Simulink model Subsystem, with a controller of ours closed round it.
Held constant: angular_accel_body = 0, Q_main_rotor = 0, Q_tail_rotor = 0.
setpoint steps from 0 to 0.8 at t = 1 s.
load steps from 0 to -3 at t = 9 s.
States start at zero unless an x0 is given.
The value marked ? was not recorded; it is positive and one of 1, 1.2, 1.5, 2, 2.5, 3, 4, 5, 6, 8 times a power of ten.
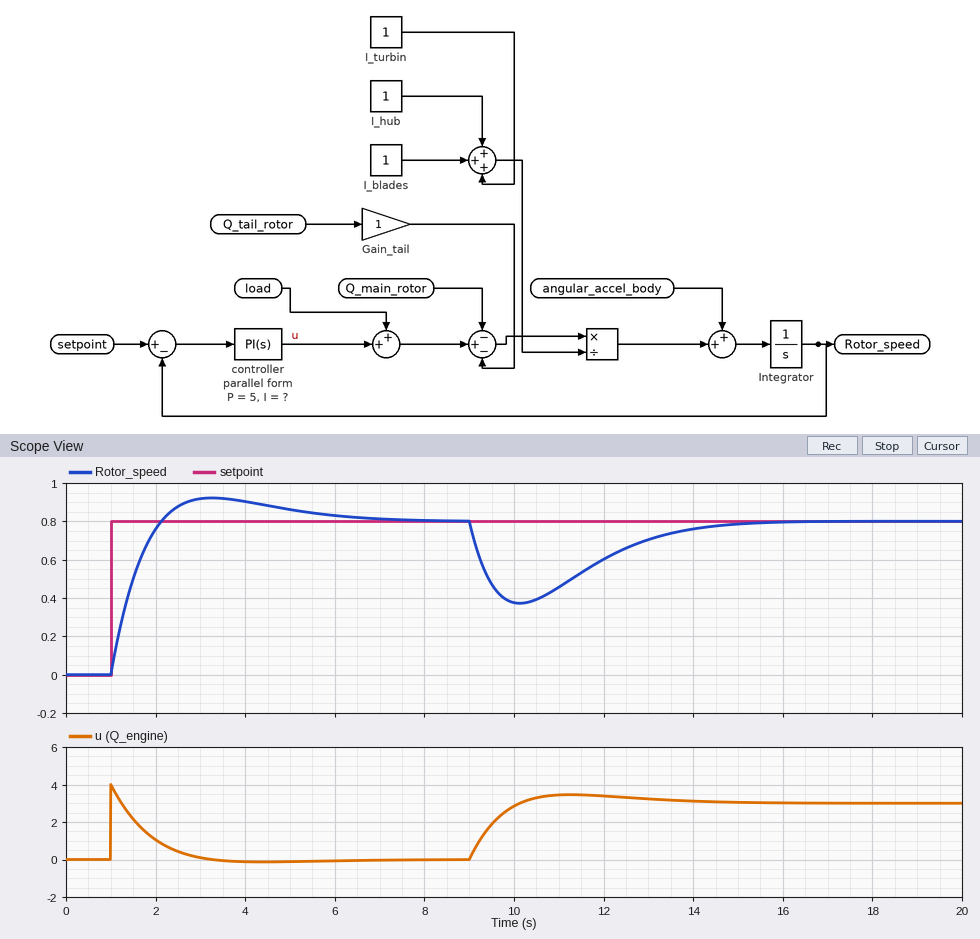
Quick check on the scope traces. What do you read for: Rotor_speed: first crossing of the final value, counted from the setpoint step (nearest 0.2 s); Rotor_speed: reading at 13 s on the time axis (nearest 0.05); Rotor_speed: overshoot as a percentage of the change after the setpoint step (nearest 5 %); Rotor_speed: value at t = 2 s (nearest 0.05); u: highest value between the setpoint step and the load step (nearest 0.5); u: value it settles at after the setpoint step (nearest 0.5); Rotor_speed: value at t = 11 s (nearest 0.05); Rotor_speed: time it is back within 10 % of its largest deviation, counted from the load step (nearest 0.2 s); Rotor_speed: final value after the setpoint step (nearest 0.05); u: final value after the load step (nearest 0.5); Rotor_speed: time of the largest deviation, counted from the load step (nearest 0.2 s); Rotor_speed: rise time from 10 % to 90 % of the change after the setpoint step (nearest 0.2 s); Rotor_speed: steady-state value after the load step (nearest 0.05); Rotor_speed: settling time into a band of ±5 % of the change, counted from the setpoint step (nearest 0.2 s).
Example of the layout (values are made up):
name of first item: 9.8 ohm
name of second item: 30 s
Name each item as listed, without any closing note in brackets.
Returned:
Rotor_speed: first crossing of the final value, counted from the setpoint step: 1.2 s
Rotor_speed: reading at 13 s on the time axis: 0.70
Rotor_speed: overshoot as a percentage of the change after the setpoint step: 15 %
Rotor_speed: value at t = 2 s: 0.75
u: highest value between the setpoint step and the load step: 4.0
u: value it settles at after the setpoint step: 0.0
Rotor_speed: value at t = 11 s: 0.45
Rotor_speed: time it is back within 10 % of its largest deviation, counted from the load step: 5.0 s
Rotor_speed: final value after the setpoint step: 0.80
u: final value after the load step: 3.0
Rotor_speed: time of the largest deviation, counted from the load step: 1.2 s
Rotor_speed: rise time from 10 % to 90 % of the change after the setpoint step: 0.8 s
Rotor_speed: steady-state value after the load step: 0.80
Rotor_speed: settling time into a band of ±5 % of the change, counted from the setpoint step: 4.6 s
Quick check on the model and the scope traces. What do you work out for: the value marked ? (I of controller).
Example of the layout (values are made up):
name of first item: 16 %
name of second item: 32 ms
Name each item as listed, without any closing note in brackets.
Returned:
the value marked ?: 2.5
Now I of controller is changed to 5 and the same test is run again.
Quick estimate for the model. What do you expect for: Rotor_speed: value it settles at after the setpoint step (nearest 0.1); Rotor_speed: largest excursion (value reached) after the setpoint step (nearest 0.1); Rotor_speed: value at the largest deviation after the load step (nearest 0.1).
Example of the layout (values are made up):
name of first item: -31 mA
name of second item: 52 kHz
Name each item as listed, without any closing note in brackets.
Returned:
Rotor_speed: value it settles at after the setpoint step: 0.8
Rotor_speed: largest excursion (value reached) after the setpoint step: 1.0
Rotor_speed: value at the largest deviation after the load step: 0.4
